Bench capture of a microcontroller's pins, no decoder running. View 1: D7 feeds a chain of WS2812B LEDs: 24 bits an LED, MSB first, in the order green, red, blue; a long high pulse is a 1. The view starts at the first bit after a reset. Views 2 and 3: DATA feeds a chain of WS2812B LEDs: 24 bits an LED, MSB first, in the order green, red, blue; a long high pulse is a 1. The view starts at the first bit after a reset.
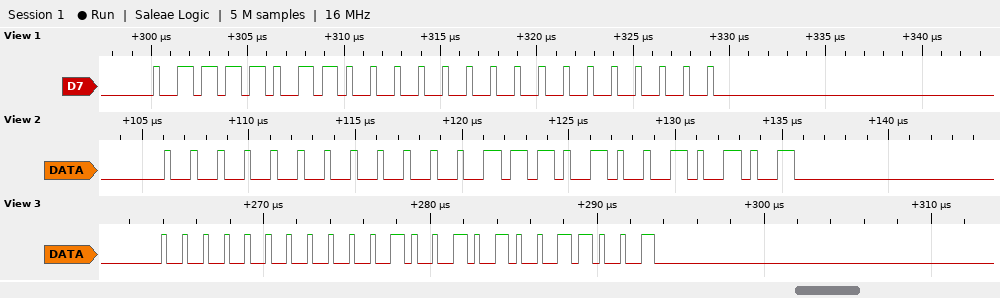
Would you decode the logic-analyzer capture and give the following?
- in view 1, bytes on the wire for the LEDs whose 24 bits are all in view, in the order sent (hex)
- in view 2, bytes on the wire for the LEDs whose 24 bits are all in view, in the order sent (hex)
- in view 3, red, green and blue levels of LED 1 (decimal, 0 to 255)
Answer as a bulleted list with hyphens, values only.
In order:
- 7B 00 00
- 00 0E 95
- 18, 0, 153
